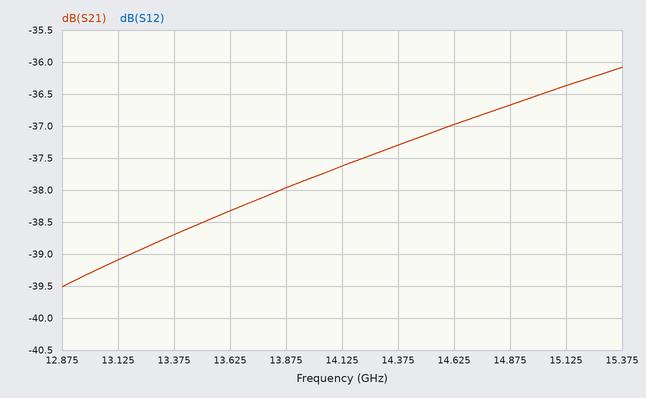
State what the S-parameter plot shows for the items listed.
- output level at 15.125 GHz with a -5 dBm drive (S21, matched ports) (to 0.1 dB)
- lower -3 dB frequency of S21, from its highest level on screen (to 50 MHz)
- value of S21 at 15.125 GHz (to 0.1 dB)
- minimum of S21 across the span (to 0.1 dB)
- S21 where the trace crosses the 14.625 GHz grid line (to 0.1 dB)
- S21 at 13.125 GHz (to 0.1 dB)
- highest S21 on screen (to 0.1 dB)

-41.4 dBm
13.15 GHz
-36.4 dB
-39.5 dB
-37.0 dB
-39.1 dB
-36.1 dB
